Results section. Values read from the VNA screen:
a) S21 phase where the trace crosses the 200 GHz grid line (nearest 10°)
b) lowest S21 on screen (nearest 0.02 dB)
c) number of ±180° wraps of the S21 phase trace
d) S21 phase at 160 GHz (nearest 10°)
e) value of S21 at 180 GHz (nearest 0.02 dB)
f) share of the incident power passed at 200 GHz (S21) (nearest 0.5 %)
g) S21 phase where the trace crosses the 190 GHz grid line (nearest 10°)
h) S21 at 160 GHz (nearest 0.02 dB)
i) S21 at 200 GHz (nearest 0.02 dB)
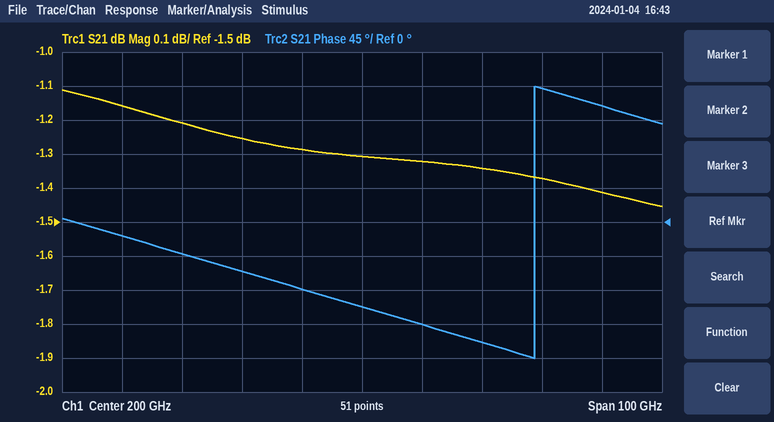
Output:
-110°
-1.46 dB
1
-20°
-1.26 dB
74.0 %
-90°
-1.16 dB
-1.30 dB
